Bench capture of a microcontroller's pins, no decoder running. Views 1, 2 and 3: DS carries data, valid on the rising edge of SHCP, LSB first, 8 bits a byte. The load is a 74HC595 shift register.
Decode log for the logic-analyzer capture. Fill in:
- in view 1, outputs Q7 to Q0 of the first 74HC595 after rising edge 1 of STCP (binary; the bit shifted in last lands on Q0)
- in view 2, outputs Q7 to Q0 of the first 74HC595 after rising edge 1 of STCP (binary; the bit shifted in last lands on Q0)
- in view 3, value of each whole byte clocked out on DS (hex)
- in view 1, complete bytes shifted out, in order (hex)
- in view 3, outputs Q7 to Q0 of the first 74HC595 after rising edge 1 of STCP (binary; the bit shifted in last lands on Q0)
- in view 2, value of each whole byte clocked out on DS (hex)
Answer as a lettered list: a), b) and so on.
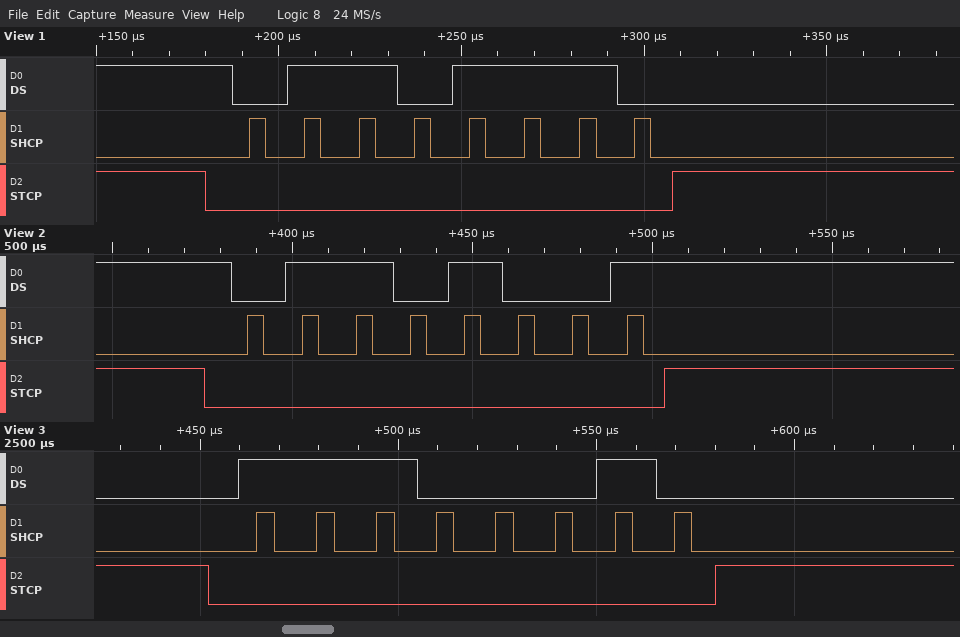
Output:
a) 01101110
b) 01101001
c) 47
d) 76
e) 11100010
f) 96
